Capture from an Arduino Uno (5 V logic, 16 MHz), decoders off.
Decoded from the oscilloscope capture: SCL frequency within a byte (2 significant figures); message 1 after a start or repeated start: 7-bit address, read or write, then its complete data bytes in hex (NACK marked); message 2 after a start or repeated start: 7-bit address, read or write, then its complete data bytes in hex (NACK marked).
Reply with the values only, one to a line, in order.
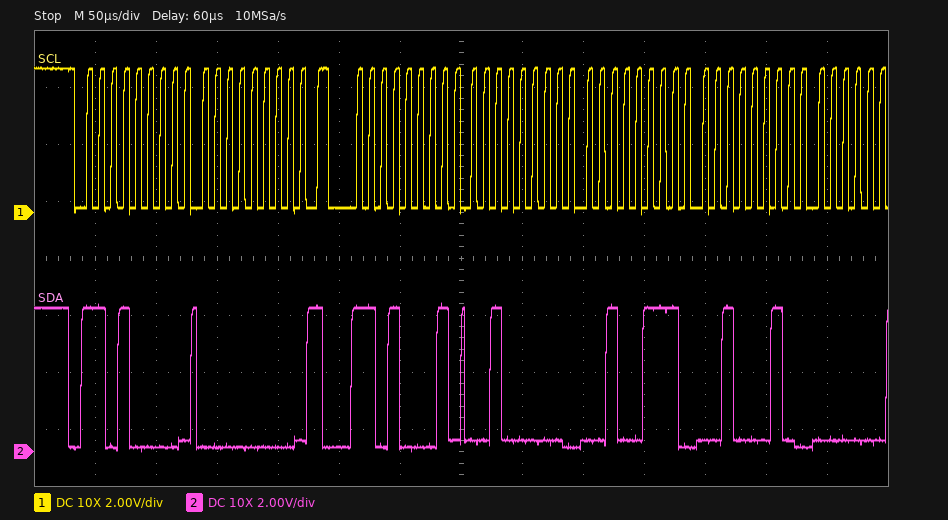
100 kHz
0x68 write: 00
0x68 read: 20 27 22
